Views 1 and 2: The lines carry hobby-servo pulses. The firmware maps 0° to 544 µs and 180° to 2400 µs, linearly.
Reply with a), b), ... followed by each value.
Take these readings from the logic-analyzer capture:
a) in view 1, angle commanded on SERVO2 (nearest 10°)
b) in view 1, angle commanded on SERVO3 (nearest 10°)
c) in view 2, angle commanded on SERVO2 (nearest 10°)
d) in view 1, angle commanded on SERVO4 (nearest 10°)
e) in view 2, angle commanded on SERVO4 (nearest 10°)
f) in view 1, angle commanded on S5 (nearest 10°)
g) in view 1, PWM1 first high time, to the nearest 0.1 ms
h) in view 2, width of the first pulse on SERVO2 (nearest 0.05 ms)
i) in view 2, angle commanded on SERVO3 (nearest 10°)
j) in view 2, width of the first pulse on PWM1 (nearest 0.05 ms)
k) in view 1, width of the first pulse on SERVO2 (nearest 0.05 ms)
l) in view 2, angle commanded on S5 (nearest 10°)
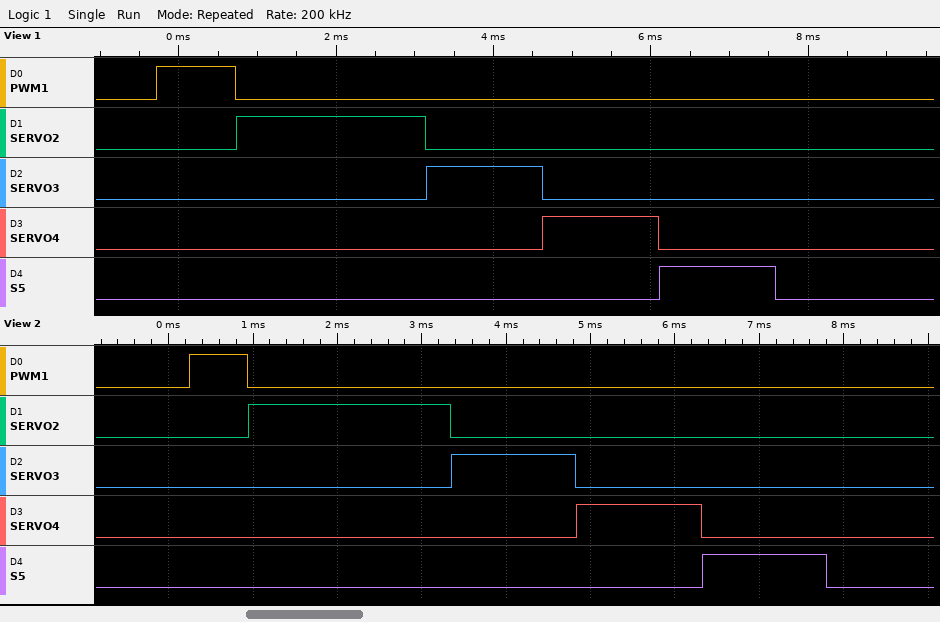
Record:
a) 180°
b) 90°
c) 180°
d) 90°
e) 90°
f) 90°
g) 1.0 ms
h) 2.40 ms
i) 90°
j) 0.70 ms
k) 2.40 ms
l) 90°
